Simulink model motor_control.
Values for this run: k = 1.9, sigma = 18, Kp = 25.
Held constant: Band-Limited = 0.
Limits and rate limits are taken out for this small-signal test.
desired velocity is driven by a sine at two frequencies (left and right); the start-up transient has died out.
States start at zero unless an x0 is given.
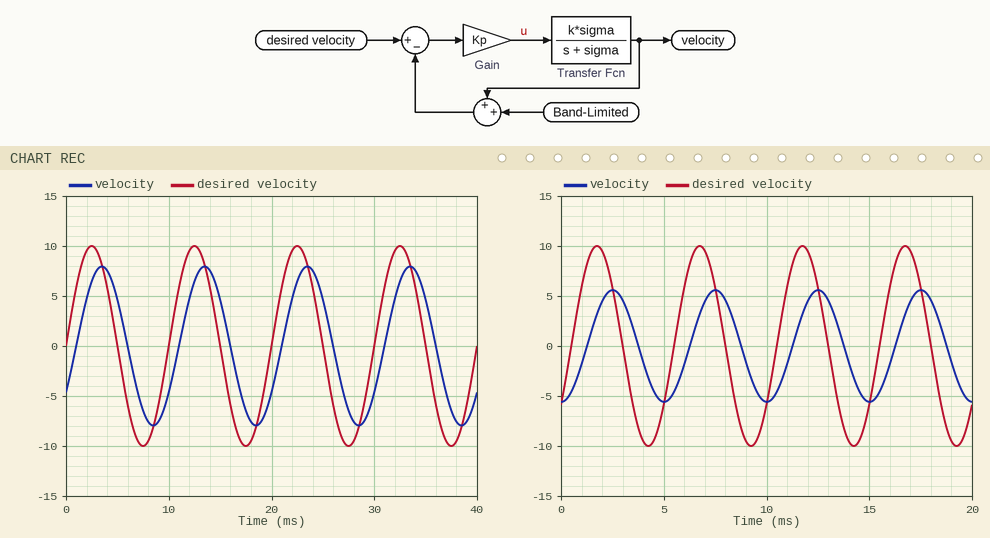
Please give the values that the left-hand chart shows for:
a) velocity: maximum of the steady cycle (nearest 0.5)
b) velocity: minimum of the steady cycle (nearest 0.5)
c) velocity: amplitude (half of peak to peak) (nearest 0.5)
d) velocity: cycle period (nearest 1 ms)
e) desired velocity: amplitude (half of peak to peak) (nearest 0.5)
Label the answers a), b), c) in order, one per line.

a) 8.0
b) -8.0
c) 8.0
d) 10 ms
e) 10.0
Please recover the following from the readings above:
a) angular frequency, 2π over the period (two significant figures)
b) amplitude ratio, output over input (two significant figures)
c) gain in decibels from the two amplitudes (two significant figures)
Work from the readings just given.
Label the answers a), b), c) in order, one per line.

a) 0.63 rad/ms
b) 0.80
c) -1.9 dB
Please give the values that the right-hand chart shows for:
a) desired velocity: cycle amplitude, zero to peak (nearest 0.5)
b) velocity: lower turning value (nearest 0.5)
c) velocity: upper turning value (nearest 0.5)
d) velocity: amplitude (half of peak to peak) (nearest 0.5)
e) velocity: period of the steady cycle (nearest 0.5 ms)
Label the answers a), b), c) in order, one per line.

a) 10.0
b) -5.5
c) 5.5
d) 5.5
e) 5.0 ms
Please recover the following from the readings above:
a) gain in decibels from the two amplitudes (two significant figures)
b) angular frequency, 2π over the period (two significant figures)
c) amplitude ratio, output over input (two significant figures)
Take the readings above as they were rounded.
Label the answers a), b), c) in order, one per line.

a) -5.2 dB
b) 1.3 rad/ms
c) 0.55
